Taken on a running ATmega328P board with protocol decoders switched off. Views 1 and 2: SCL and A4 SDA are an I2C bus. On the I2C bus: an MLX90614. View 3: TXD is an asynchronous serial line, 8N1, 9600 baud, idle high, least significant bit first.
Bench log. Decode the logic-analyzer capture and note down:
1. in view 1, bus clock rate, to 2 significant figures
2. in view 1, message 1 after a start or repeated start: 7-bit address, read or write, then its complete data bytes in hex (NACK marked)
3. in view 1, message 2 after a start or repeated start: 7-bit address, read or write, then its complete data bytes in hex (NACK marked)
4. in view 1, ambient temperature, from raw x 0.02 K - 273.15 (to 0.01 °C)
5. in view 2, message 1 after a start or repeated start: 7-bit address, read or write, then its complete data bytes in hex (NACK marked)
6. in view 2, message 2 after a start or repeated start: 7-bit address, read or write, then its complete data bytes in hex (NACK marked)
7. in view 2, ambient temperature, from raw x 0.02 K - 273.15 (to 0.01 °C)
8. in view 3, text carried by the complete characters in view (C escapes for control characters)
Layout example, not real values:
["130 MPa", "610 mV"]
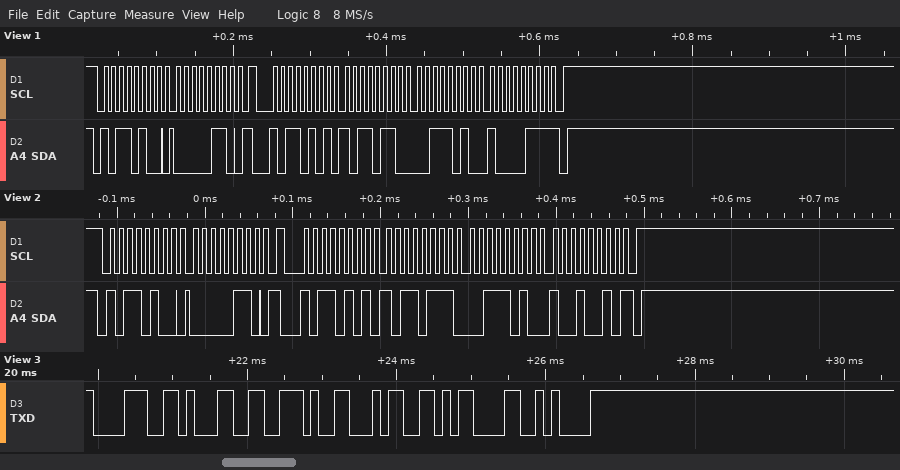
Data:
["100 kHz", "0x5A write: 06", "0x5A read: B6 3A 87 NACK", "27.45 °C", "0x5A write: 06", "0x5A read: B7 3A 92 NACK", "27.47 °C", "\"81.4\\r\\n\""]
